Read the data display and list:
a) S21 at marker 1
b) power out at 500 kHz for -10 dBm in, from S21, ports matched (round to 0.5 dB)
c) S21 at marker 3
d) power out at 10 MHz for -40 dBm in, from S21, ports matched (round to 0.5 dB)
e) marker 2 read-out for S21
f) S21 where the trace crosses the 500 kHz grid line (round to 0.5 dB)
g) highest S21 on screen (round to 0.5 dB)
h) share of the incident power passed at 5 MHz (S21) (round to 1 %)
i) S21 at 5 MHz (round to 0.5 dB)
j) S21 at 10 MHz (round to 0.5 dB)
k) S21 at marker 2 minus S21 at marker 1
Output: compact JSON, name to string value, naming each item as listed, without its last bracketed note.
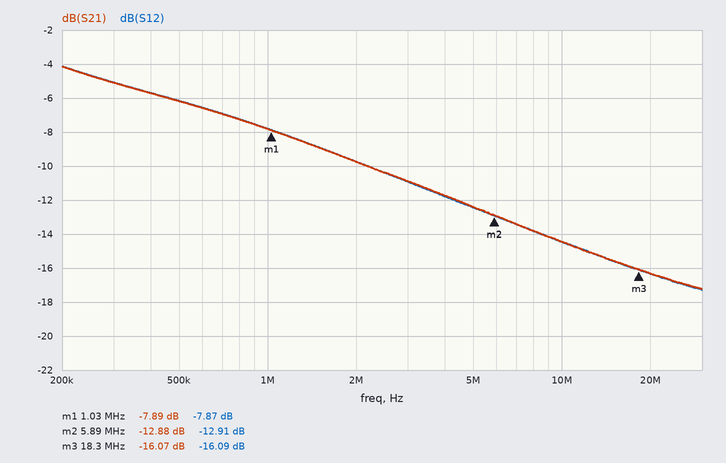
{"S21 at marker 1": "-7.89 dB", "power out at 500 kHz for -10 dBm in, from S21, ports matched": "-16.0 dBm", "S21 at marker 3": "-16.07 dB", "power out at 10 MHz for -40 dBm in, from S21, ports matched": "-54.5 dBm", "marker 2 read-out for S21": "-12.88 dB", "S21 where the trace crosses the 500 kHz grid line": "-6.0 dB", "highest S21 on screen": "-4.0 dB", "share of the incident power passed at 5 MHz (S21)": "6 %", "S21 at 5 MHz": "-12.5 dB", "S21 at 10 MHz": "-14.5 dB", "S21 at marker 2 minus S21 at marker 1": "-4.99 dB"}
